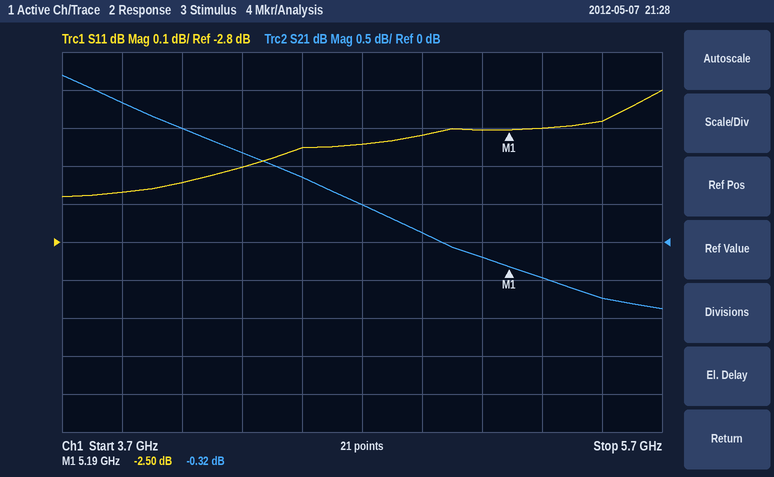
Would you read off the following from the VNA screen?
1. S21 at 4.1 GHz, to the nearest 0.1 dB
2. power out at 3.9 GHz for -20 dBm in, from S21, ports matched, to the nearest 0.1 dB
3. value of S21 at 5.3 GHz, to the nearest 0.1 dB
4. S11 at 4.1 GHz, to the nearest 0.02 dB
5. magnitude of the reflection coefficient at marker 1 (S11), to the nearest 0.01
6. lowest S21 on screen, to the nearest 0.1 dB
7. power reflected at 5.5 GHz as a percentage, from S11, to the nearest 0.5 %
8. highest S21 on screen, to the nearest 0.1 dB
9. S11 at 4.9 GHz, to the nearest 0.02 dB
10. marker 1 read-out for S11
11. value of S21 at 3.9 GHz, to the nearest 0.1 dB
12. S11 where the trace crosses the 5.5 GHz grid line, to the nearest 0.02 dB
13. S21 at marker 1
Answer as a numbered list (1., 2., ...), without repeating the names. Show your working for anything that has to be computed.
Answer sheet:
1. 1.5 dB
2. -20 dBm + (1.8 dB) = -18.2 dBm
3. -0.5 dB
4. -2.64 dB
5. 10^(-2.5/20) ≈ 0.75
6. -0.9 dB
7. 10^(-2.48/10) ≈ 56.5 %
8. 2.2 dB
9. -2.52 dB
10. -2.50 dB
11. 1.8 dB
12. -2.48 dB
13. -0.32 dB
